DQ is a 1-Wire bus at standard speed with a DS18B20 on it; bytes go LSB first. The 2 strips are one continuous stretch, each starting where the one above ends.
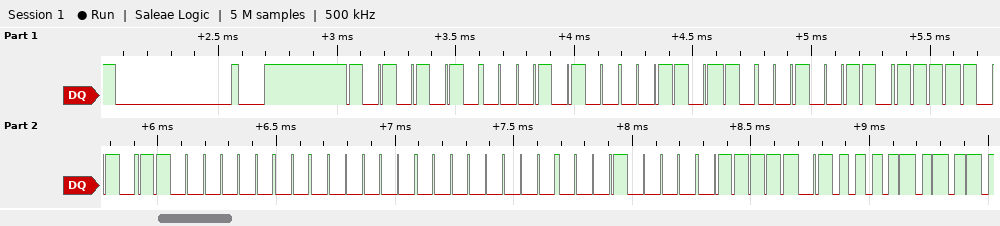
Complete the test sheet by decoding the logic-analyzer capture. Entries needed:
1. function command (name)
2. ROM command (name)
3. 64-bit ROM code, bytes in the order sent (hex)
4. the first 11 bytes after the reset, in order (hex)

Read Scratchpad
Match ROM
28 6C 64 5F 03 00 00 08
55 28 6C 64 5F 03 00 00 08 BE 50
